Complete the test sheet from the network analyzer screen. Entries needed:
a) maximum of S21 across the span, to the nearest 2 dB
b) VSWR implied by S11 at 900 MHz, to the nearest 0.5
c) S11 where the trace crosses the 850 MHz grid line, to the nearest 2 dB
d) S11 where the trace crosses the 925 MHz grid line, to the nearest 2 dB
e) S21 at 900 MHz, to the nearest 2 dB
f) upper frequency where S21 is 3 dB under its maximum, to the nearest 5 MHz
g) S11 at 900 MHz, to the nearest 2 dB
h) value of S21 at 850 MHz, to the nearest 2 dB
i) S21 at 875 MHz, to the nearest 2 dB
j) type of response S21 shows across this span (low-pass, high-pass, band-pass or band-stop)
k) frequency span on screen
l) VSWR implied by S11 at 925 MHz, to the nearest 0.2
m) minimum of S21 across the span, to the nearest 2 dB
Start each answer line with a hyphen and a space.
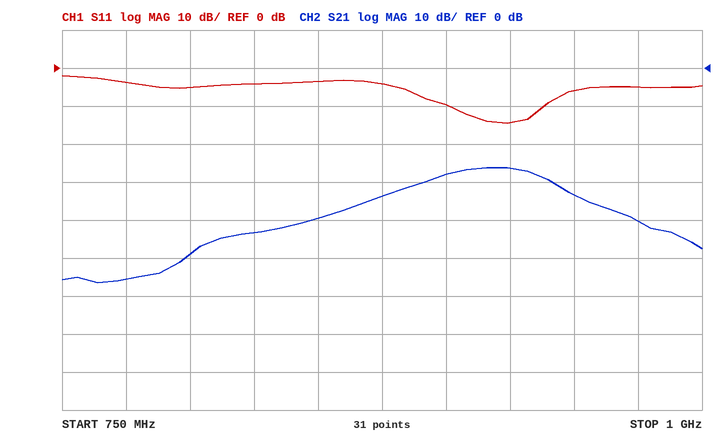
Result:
- -26 dB
- 2.0
- -4 dB
- -14 dB
- -28 dB
- 940 MHz
- -10 dB
- -40 dB
- -34 dB
- band-pass
- 250 MHz
- 1.4
- -56 dB
